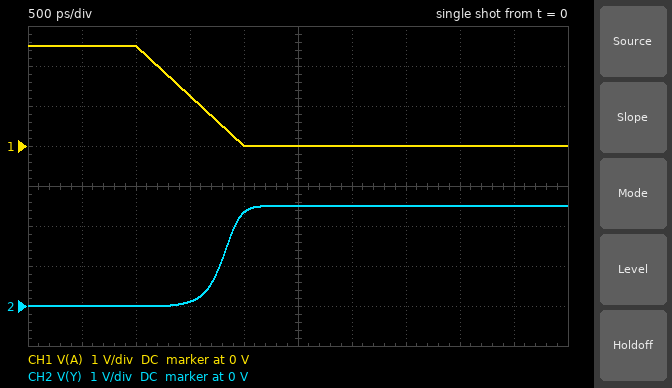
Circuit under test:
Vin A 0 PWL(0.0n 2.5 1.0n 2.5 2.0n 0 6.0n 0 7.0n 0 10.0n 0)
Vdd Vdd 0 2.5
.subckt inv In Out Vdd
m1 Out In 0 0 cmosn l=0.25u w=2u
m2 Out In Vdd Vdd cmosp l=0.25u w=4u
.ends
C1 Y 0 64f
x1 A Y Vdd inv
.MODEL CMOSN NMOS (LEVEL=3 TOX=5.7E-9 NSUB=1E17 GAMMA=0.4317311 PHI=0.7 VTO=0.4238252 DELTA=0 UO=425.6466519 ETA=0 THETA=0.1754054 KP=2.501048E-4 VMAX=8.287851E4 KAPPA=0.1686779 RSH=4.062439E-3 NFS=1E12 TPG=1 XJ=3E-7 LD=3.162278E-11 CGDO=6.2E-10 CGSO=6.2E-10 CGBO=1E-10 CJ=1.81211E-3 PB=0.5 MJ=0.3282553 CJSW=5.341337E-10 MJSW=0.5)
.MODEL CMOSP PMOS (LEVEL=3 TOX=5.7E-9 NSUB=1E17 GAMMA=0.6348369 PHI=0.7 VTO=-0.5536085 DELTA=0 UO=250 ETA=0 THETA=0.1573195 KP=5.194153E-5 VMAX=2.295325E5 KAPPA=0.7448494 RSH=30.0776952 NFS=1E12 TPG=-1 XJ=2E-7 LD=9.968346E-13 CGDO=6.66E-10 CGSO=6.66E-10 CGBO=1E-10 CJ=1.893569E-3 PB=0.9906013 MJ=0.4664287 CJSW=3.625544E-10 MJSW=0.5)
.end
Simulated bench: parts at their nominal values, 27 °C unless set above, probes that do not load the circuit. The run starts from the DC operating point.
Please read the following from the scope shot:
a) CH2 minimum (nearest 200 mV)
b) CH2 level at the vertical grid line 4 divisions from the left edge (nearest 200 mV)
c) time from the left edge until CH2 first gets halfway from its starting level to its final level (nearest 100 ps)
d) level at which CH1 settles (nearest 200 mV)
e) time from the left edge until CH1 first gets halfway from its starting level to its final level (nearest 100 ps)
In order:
0 V
2.4 V
1.8 ns
0 V
1.5 ns
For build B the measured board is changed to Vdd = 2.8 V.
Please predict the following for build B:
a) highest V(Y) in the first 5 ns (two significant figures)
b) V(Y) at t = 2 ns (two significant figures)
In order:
2.8 V
2.7 V
